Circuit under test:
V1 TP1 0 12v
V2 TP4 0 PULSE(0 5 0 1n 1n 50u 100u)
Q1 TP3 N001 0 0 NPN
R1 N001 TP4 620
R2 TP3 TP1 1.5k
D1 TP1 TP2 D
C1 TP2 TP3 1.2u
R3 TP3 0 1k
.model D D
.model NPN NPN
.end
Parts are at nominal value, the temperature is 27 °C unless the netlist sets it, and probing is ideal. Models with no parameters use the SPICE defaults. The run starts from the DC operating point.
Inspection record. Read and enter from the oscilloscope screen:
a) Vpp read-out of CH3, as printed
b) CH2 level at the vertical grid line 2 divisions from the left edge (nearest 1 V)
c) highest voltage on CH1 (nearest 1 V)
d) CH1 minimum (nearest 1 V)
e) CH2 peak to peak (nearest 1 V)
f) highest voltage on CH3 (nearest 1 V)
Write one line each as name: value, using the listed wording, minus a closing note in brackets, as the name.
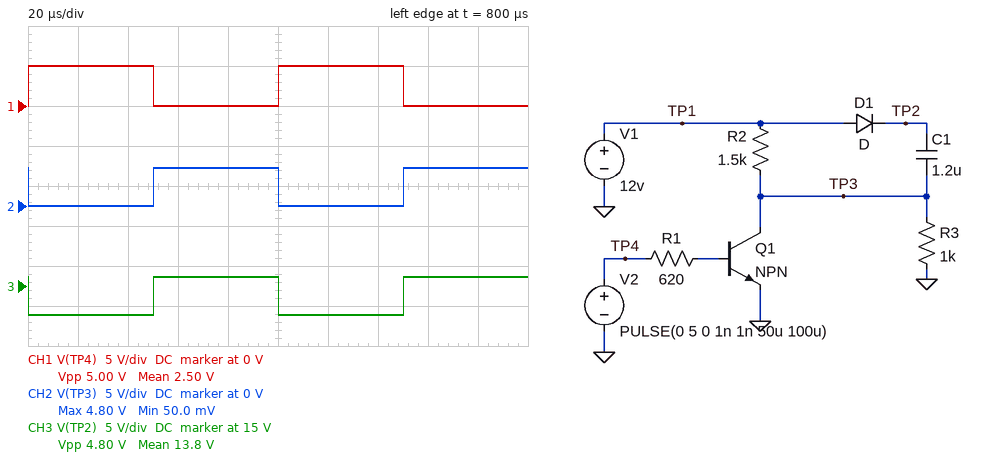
Vpp read-out of CH3, as printed: 4.80 V
CH2 level at the vertical grid line 2 divisions from the left edge: 0 V
highest voltage on CH1: 5 V
CH1 minimum: 0 V
CH2 peak to peak: 5 V
highest voltage on CH3: 16 V
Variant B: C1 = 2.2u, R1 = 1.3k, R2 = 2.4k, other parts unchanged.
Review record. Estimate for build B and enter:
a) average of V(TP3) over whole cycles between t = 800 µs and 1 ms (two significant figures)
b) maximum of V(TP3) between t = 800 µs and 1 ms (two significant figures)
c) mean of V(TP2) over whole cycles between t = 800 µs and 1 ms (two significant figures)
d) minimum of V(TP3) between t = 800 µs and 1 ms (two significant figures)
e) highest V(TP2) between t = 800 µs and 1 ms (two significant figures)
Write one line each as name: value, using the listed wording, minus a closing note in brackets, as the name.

average of V(TP3) over whole cycles between t = 800 µs and 1 ms: 1.8 V
maximum of V(TP3) between t = 800 µs and 1 ms: 3.5 V
mean of V(TP2) over whole cycles between t = 800 µs and 1 ms: 13 V
minimum of V(TP3) between t = 800 µs and 1 ms: 33 mV
highest V(TP2) between t = 800 µs and 1 ms: 15 V
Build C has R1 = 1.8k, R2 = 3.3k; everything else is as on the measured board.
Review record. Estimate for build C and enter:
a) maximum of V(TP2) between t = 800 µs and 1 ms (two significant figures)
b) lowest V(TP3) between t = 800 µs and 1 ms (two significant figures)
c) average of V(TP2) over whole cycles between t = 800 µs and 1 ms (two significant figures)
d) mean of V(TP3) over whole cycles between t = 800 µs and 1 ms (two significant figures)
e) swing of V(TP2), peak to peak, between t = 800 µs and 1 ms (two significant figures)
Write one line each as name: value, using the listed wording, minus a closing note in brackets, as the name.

maximum of V(TP2) between t = 800 µs and 1 ms: 14 V
lowest V(TP3) between t = 800 µs and 1 ms: 33 mV
average of V(TP2) over whole cycles between t = 800 µs and 1 ms: 13 V
mean of V(TP3) over whole cycles between t = 800 µs and 1 ms: 1.4 V
swing of V(TP2), peak to peak, between t = 800 µs and 1 ms: 2.8 V
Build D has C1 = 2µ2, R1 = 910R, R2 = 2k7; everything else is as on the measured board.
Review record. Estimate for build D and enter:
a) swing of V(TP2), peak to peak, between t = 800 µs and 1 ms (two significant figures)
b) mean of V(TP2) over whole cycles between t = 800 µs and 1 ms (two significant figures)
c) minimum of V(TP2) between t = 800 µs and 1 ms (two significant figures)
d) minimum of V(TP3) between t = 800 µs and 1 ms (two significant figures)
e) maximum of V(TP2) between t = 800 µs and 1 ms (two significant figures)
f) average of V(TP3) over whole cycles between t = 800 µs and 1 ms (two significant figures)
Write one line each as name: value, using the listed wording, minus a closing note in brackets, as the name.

swing of V(TP2), peak to peak, between t = 800 µs and 1 ms: 3.2 V
mean of V(TP2) over whole cycles between t = 800 µs and 1 ms: 13 V
minimum of V(TP2) between t = 800 µs and 1 ms: 11 V
minimum of V(TP3) between t = 800 µs and 1 ms: 29 mV
maximum of V(TP2) between t = 800 µs and 1 ms: 15 V
average of V(TP3) over whole cycles between t = 800 µs and 1 ms: 1.6 V
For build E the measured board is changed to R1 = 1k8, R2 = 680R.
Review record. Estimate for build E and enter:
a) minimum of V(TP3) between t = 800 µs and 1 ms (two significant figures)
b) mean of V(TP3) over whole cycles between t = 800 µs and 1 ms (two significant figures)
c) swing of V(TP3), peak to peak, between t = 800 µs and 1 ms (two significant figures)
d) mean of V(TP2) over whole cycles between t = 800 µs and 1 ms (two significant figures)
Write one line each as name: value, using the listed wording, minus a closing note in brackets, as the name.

minimum of V(TP3) between t = 800 µs and 1 ms: 61 mV
mean of V(TP3) over whole cycles between t = 800 µs and 1 ms: 3.6 V
swing of V(TP3), peak to peak, between t = 800 µs and 1 ms: 7.1 V
mean of V(TP2) over whole cycles between t = 800 µs and 1 ms: 15 V
